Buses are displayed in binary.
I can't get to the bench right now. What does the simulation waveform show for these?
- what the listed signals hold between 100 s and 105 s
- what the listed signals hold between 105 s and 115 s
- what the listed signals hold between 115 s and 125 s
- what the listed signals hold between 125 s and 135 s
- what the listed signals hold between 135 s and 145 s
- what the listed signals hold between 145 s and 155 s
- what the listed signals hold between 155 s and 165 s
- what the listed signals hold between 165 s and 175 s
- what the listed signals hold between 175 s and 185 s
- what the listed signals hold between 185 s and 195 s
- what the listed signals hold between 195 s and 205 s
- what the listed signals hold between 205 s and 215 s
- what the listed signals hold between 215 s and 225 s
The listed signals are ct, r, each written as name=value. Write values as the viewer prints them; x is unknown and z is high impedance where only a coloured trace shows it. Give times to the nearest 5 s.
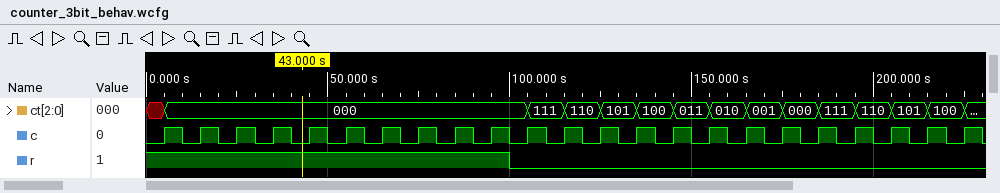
ct=000, r=0
ct=111, r=0
ct=110, r=0
ct=101, r=0
ct=100, r=0
ct=011, r=0
ct=010, r=0
ct=001, r=0
ct=000, r=0
ct=111, r=0
ct=110, r=0
ct=101, r=0
ct=100, r=0
